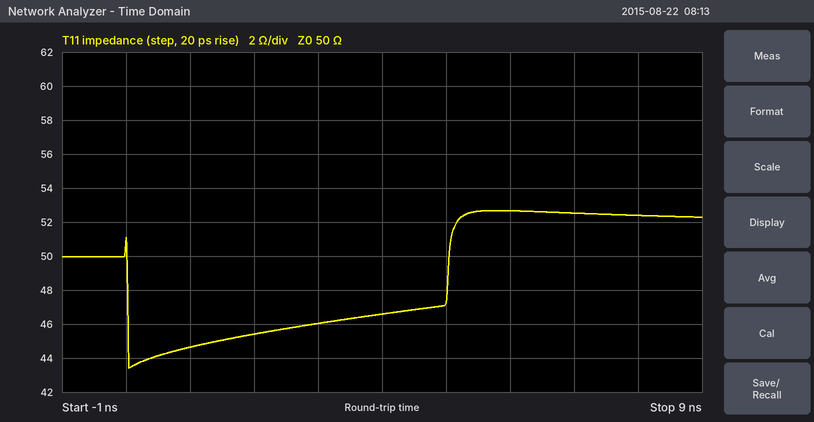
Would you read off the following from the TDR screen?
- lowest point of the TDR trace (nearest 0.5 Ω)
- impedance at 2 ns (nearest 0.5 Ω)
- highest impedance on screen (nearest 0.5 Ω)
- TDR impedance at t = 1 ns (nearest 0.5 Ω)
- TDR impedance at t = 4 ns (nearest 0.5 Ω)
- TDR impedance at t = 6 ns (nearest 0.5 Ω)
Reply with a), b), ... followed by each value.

a) 43.5 Ω
b) 45.5 Ω
c) 52.5 Ω
d) 44.5 Ω
e) 46.5 Ω
f) 52.5 Ω
